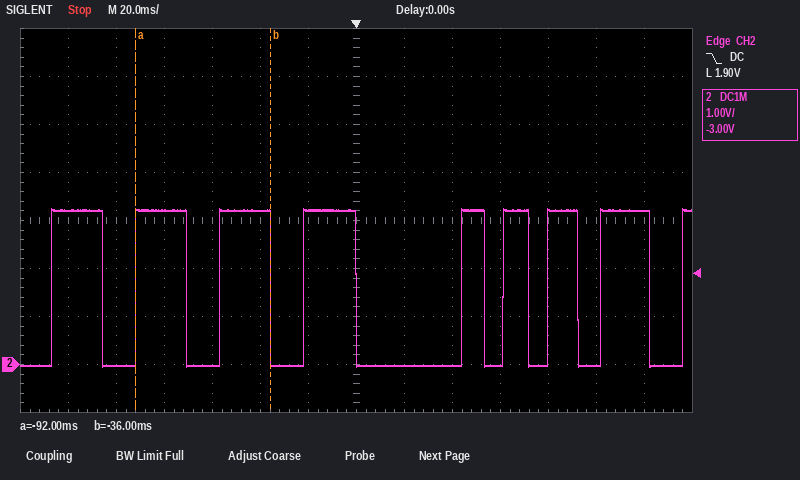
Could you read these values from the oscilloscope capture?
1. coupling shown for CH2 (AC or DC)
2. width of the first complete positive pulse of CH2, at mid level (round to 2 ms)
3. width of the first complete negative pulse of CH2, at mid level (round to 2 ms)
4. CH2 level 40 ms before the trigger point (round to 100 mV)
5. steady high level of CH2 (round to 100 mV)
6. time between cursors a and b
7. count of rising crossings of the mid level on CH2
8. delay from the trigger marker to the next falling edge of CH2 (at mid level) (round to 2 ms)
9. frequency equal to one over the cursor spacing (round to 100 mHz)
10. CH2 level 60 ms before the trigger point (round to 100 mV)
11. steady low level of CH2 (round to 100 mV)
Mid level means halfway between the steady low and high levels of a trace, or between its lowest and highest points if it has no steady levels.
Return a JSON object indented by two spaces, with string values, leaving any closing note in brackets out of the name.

{
  "coupling shown for CH2": "DC",
  "width of the first complete positive pulse of CH2, at mid level": "22 ms",
  "width of the first complete negative pulse of CH2, at mid level": "14 ms",
  "CH2 level 40 ms before the trigger point": "3.2 V",
  "steady high level of CH2": "3.2 V",
  "time between cursors a and b": "56 ms",
  "count of rising crossings of the mid level on CH2": "9",
  "delay from the trigger marker to the next falling edge of CH2 (at mid level)": "54 ms",
  "frequency equal to one over the cursor spacing": "17.9 Hz",
  "CH2 level 60 ms before the trigger point": "0.0 V",
  "steady low level of CH2": "0.0 V"
}
